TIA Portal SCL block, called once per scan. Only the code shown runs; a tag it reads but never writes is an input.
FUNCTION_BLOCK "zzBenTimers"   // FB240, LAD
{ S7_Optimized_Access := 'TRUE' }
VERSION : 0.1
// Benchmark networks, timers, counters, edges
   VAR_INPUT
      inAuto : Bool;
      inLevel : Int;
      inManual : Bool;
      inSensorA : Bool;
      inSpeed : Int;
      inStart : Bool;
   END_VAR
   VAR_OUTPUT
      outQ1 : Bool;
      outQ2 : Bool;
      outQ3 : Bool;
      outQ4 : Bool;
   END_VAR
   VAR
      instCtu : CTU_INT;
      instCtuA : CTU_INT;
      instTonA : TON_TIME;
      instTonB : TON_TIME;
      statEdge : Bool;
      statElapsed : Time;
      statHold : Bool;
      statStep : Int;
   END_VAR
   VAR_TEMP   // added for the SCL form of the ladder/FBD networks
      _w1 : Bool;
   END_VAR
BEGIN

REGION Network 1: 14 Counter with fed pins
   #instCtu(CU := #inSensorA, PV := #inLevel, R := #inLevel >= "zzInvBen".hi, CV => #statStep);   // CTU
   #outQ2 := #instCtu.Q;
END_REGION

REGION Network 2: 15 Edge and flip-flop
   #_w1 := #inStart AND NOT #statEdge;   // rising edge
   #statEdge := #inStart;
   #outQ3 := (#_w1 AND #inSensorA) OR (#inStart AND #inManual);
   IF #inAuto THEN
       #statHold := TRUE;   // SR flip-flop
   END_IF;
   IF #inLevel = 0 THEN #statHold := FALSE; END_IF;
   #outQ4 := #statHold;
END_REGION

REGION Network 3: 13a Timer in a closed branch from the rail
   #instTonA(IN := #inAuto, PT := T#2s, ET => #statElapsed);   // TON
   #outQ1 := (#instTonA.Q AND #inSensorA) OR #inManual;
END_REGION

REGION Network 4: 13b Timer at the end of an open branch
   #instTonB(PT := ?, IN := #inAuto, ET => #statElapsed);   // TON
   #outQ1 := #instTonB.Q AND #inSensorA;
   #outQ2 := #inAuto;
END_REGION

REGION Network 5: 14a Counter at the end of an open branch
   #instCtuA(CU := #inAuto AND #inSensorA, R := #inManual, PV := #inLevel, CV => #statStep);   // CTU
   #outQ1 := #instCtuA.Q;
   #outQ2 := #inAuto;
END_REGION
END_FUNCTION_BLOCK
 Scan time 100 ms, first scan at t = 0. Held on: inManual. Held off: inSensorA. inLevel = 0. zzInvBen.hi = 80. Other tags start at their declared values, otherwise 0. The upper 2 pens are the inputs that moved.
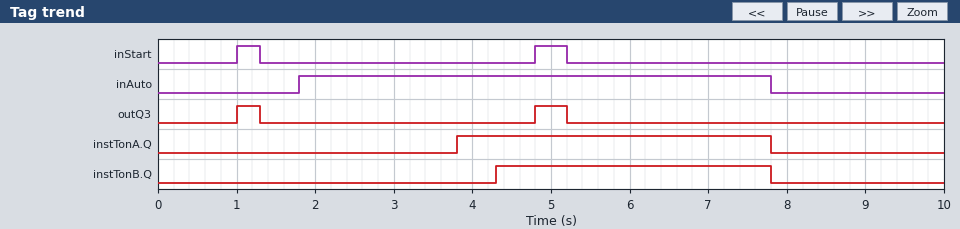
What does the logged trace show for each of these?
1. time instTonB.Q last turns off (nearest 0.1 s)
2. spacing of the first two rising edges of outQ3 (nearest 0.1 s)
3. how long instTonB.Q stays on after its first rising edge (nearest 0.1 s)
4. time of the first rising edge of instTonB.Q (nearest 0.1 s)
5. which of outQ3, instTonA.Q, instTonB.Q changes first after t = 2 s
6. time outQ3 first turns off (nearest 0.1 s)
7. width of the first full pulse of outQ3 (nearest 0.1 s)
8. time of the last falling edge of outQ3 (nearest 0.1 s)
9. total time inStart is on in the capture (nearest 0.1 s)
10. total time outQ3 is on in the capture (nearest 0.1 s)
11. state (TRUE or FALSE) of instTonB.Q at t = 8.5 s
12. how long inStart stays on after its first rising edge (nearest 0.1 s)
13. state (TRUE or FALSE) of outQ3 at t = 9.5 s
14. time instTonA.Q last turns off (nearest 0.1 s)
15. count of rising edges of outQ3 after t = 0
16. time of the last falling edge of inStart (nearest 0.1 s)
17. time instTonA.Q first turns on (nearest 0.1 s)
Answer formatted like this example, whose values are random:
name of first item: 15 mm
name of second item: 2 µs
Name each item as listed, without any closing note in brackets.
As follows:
time instTonB.Q last turns off: 7.8 s
spacing of the first two rising edges of outQ3: 3.8 s
how long instTonB.Q stays on after its first rising edge: 3.5 s
time of the first rising edge of instTonB.Q: 4.3 s
which of outQ3, instTonA.Q, instTonB.Q changes first after t = 2 s: instTonA.Q
time outQ3 first turns off: 1.3 s
width of the first full pulse of outQ3: 0.3 s
time of the last falling edge of outQ3: 5.2 s
total time inStart is on in the capture: 0.7 s
total time outQ3 is on in the capture: 0.7 s
state (TRUE or FALSE) of instTonB.Q at t = 8.5 s: FALSE
how long inStart stays on after its first rising edge: 0.3 s
state (TRUE or FALSE) of outQ3 at t = 9.5 s: FALSE
time instTonA.Q last turns off: 7.8 s
count of rising edges of outQ3 after t = 0: 2
time of the last falling edge of inStart: 5.2 s
time instTonA.Q first turns on: 3.8 s
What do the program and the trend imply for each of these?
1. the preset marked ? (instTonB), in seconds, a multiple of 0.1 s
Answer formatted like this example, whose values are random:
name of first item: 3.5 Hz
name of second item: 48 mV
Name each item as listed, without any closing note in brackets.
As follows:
the preset marked ? (instTonB), in seconds, a multiple of 0.1 s: 2.5 s
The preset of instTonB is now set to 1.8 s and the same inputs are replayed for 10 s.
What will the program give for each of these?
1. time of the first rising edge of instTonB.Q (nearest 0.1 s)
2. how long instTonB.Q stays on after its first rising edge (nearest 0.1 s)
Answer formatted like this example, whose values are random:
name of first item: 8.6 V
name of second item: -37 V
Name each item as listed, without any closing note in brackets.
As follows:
time of the first rising edge of instTonB.Q: 3.6 s
how long instTonB.Q stays on after its first rising edge: 4.2 s
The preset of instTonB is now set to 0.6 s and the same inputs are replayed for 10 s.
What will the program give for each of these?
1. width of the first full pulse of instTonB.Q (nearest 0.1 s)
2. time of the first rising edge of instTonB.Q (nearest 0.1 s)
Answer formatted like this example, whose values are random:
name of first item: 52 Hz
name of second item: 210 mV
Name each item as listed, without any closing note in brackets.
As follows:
width of the first full pulse of instTonB.Q: 5.4 s
time of the first rising edge of instTonB.Q: 2.4 s
